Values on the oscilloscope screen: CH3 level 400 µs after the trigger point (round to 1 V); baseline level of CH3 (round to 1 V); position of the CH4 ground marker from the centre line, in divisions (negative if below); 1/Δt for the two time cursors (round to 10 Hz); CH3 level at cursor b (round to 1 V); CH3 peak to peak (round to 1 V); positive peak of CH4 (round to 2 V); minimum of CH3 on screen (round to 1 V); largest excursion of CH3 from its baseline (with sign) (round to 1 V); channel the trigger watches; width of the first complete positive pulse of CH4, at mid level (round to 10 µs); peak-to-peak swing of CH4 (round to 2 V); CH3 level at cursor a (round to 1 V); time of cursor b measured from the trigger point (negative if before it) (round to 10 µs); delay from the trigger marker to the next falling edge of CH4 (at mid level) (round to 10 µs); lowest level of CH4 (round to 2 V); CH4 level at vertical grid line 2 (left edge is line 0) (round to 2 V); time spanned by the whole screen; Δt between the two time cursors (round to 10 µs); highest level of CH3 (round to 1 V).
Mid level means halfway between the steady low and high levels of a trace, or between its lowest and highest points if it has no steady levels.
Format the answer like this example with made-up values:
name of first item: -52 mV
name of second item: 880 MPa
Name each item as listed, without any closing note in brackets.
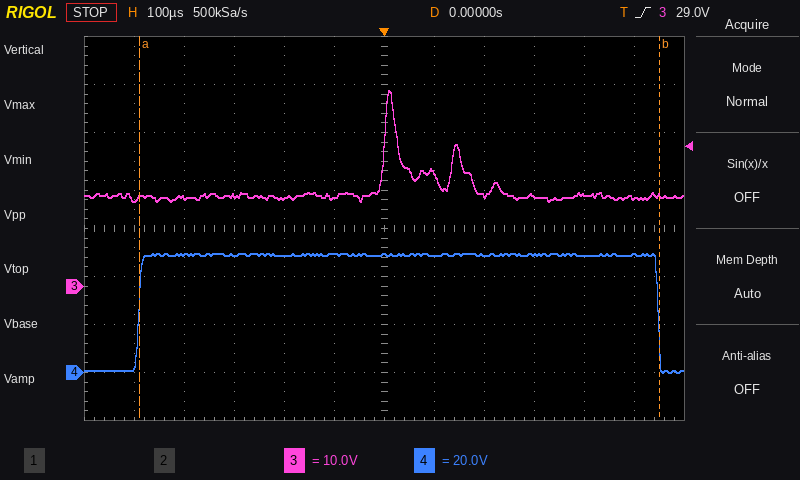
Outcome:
CH3 level 400 µs after the trigger point: 19 V
baseline level of CH3: 19 V
position of the CH4 ground marker from the centre line, in divisions: -3.0 div
1/Δt for the two time cursors: 960 Hz
CH3 level at cursor b: 19 V
CH3 peak to peak: 23 V
positive peak of CH4: 50 V
minimum of CH3 on screen: 18 V
largest excursion of CH3 from its baseline (with sign): +22 V
channel the trigger watches: CH3
width of the first complete positive pulse of CH4, at mid level: 1.04 ms
peak-to-peak swing of CH4: 50 V
CH3 level at cursor a: 18 V
time of cursor b measured from the trigger point (negative if before it): +550 µs
delay from the trigger marker to the next falling edge of CH4 (at mid level): 550 µs
lowest level of CH4: 0 V
CH4 level at vertical grid line 2 (left edge is line 0): 50 V
time spanned by the whole screen: 1.2 ms
Δt between the two time cursors: 1.04 ms
highest level of CH3: 41 V
